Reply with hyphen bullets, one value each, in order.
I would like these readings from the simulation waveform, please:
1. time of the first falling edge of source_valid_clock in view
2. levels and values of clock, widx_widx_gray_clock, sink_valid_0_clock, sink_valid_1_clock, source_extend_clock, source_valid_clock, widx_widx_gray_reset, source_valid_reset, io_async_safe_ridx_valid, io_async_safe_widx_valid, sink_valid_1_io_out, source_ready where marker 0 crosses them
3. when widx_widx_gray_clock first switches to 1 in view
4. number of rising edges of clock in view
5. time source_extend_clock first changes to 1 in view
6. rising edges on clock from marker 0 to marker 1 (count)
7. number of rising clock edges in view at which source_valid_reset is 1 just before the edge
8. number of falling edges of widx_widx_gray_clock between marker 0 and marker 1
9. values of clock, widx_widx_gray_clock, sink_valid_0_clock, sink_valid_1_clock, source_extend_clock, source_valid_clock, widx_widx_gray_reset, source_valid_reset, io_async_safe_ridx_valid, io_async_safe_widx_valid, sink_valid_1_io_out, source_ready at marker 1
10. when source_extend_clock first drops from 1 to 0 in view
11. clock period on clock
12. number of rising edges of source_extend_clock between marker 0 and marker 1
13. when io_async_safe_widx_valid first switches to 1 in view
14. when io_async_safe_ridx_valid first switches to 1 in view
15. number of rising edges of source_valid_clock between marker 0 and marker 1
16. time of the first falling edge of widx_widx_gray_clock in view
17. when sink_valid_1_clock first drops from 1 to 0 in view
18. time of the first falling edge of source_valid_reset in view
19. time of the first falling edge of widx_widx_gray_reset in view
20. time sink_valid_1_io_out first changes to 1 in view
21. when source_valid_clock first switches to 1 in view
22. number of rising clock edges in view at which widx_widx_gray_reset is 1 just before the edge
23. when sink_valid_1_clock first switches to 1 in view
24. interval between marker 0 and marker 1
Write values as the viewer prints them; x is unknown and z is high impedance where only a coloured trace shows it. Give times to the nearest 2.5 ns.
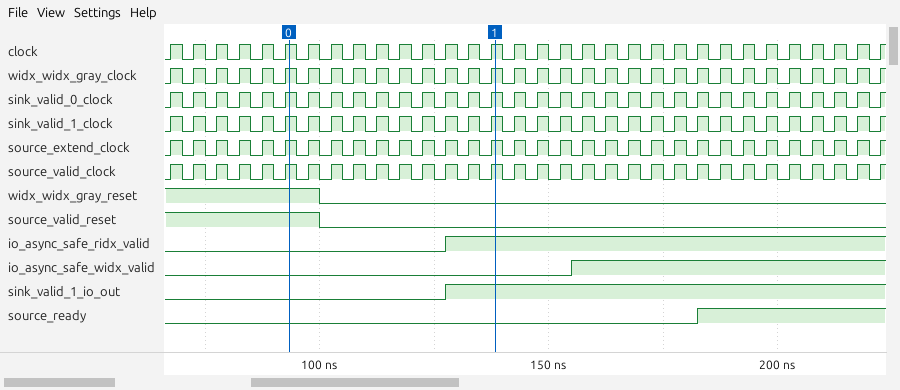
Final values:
- 70 ns
- clock=1, widx_widx_gray_clock=1, sink_valid_0_clock=1, sink_valid_1_clock=1, source_extend_clock=1, source_valid_clock=1, widx_widx_gray_reset=1, source_valid_reset=1, io_async_safe_ridx_valid=0, io_async_safe_widx_valid=0, sink_valid_1_io_out=0, source_ready=0
- 67.5 ns
- 32
- 67.5 ns
- 9
- 7
- 9
- clock=1, widx_widx_gray_clock=1, sink_valid_0_clock=1, sink_valid_1_clock=1, source_extend_clock=1, source_valid_clock=1, widx_widx_gray_reset=0, source_valid_reset=0, io_async_safe_ridx_valid=1, io_async_safe_widx_valid=0, sink_valid_1_io_out=1, source_ready=0
- 70 ns
- 5 ns
- 9
- 155 ns
- 127.5 ns
- 9
- 70 ns
- 70 ns
- 100 ns
- 100 ns
- 127.5 ns
- 67.5 ns
- 7
- 67.5 ns
- 45 ns
